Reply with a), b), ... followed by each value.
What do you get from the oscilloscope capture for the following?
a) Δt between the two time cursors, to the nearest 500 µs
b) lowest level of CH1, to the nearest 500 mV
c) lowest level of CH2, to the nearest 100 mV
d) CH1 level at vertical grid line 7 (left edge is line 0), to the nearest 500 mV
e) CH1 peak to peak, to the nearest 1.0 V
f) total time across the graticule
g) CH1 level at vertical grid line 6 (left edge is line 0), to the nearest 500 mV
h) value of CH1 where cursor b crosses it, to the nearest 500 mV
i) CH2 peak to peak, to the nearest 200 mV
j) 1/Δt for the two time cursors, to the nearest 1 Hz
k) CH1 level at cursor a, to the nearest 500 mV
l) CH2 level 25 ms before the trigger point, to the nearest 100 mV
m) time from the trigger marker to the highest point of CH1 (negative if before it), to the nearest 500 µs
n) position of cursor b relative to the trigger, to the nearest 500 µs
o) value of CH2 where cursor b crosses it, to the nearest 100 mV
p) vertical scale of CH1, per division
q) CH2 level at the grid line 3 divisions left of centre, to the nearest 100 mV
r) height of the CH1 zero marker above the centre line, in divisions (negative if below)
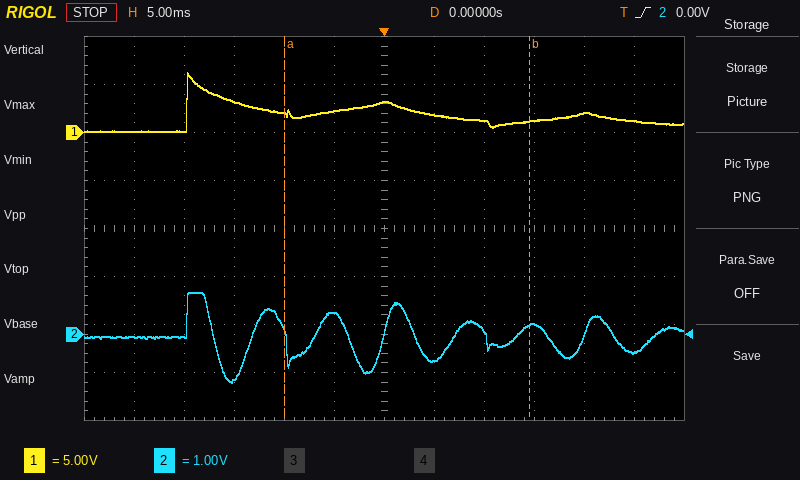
a) 24.5 ms
b) 0.0 V
c) -1.0 V
d) 2.0 V
e) 6.0 V
f) 60 ms
g) 3.0 V
h) 1.0 V
i) 1.8 V
j) 41 Hz
k) 2.0 V
l) -100 mV
m) -19.5 ms
n) +14.5 ms
o) 200 mV
p) 5 V
q) -900 mV
r) +2.0 div
